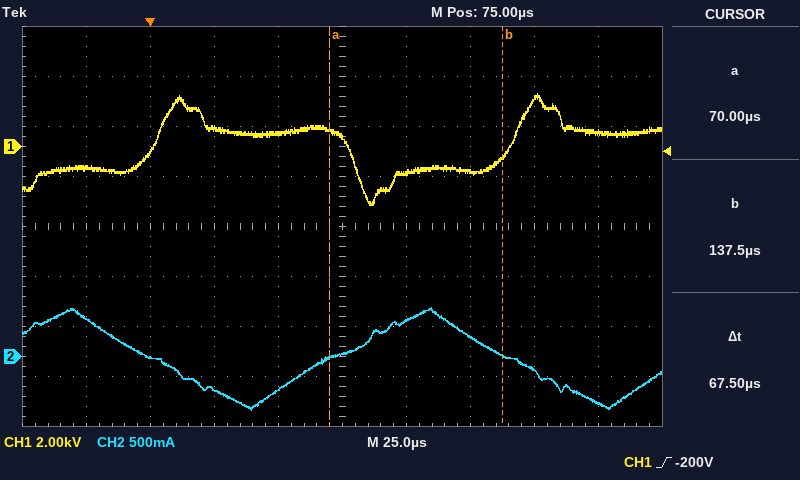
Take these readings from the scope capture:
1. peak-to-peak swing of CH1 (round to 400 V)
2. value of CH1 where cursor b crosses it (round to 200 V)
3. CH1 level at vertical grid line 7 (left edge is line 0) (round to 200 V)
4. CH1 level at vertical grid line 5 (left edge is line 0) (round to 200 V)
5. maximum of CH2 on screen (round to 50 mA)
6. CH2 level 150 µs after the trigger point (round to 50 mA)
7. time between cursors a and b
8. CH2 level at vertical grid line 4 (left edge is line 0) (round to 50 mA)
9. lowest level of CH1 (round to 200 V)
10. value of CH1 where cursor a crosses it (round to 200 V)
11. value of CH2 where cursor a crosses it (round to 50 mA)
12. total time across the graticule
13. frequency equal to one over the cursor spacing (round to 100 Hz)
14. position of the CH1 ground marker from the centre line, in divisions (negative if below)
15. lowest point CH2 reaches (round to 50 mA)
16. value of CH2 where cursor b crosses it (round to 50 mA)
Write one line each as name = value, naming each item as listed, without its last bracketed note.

peak-to-peak swing of CH1 = 4.4 kV
value of CH1 where cursor b crosses it = -400 V
CH1 level at vertical grid line 7 (left edge is line 0) = -1.0 kV
CH1 level at vertical grid line 5 (left edge is line 0) = 400 V
maximum of CH2 on screen = 500 mA
CH2 level 150 µs after the trigger point = -150 mA
time between cursors a and b = 67.5 µs
CH2 level at vertical grid line 4 (left edge is line 0) = -350 mA
lowest level of CH1 = -2.4 kV
value of CH1 where cursor a crosses it = 600 V
value of CH2 where cursor a crosses it = 0 mA
total time across the graticule = 250 µs
frequency equal to one over the cursor spacing = 14.8 kHz
position of the CH1 ground marker from the centre line, in divisions = +1.6 div
lowest point CH2 reaches = -550 mA
value of CH2 where cursor b crosses it = 0 mA
